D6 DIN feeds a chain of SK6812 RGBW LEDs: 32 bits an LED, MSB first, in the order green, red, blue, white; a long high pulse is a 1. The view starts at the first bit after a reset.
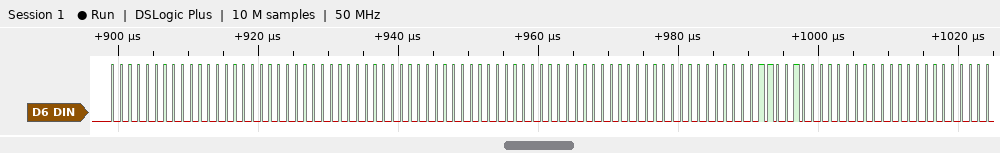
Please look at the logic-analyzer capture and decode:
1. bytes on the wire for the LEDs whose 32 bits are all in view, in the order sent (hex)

00 00 00 00 00 00 00 00 00 32 00 00
